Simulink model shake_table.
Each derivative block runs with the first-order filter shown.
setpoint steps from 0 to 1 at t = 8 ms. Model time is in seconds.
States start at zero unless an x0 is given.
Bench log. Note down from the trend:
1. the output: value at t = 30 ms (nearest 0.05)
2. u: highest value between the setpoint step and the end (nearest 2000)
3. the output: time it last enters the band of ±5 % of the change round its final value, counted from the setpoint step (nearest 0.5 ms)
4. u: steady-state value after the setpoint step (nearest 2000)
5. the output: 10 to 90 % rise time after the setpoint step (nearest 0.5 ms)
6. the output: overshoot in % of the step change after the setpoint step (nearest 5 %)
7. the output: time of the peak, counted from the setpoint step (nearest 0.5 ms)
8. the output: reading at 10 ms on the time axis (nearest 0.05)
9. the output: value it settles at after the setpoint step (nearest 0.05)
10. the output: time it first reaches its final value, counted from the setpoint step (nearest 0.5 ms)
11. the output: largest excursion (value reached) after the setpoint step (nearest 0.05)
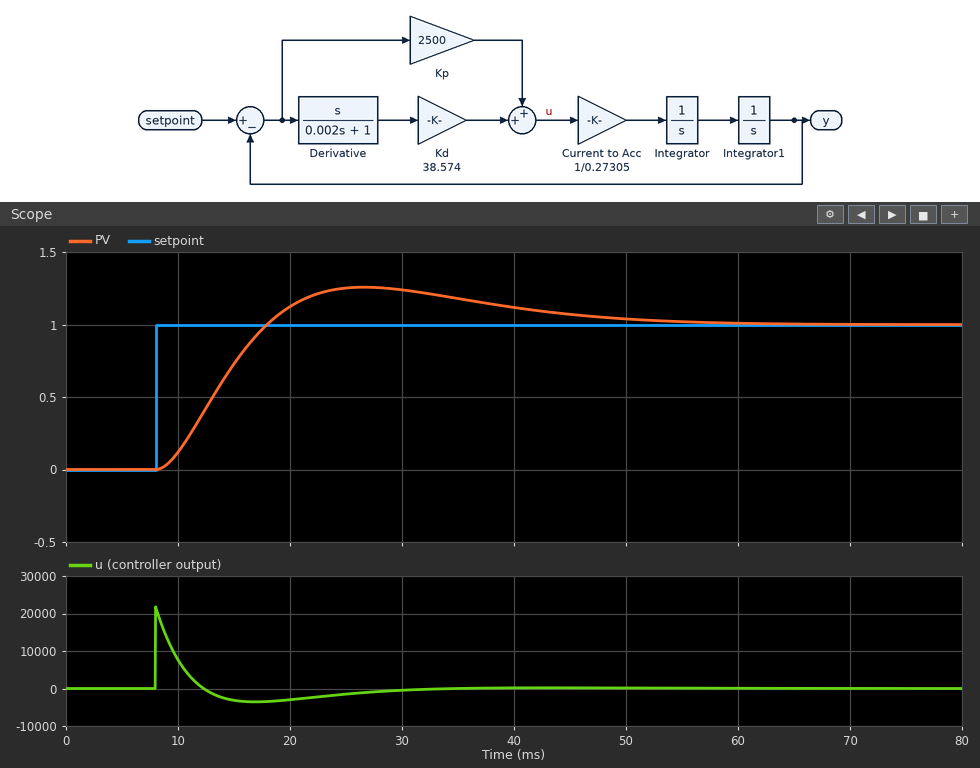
1.25
22000
40.0 ms
0
7.0 ms
25 %
18.5 ms
0.10
1.00
10.0 ms
1.25
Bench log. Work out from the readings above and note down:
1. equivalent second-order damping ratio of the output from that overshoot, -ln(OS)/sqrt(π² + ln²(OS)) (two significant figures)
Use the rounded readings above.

0.40
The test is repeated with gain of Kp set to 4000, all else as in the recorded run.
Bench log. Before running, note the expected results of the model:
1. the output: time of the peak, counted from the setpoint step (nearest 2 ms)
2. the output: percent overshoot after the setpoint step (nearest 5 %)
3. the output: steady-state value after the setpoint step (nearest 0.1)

16 ms
35 %
1.0
